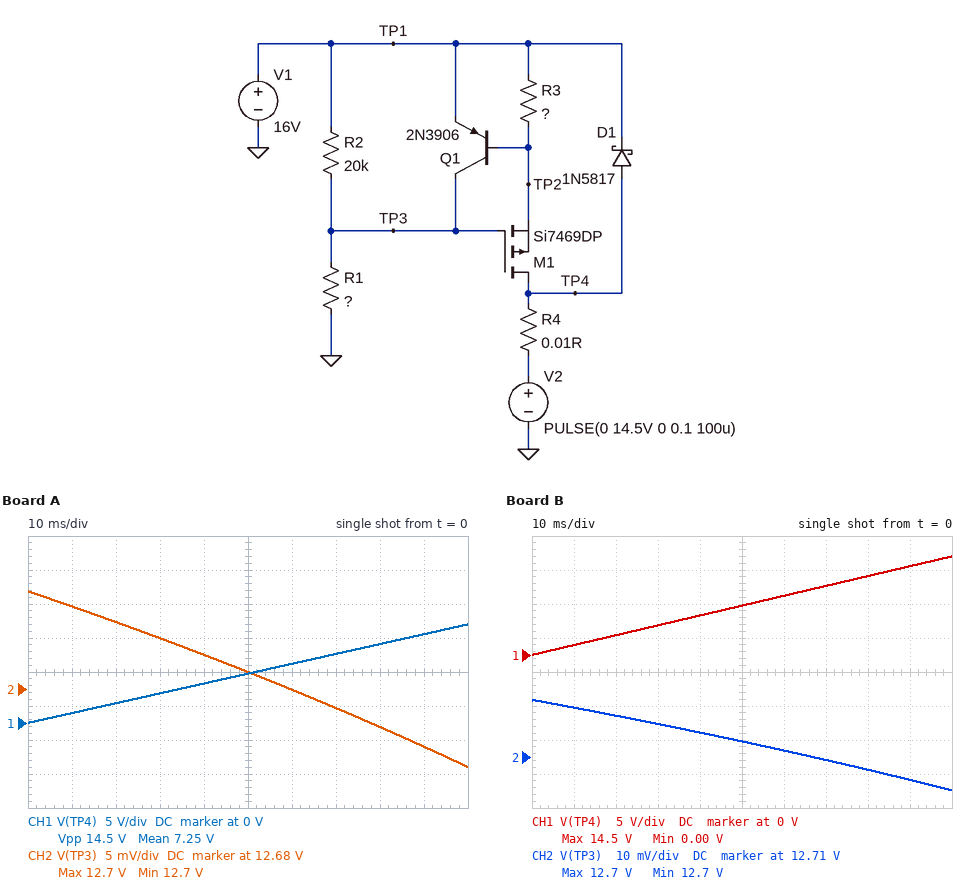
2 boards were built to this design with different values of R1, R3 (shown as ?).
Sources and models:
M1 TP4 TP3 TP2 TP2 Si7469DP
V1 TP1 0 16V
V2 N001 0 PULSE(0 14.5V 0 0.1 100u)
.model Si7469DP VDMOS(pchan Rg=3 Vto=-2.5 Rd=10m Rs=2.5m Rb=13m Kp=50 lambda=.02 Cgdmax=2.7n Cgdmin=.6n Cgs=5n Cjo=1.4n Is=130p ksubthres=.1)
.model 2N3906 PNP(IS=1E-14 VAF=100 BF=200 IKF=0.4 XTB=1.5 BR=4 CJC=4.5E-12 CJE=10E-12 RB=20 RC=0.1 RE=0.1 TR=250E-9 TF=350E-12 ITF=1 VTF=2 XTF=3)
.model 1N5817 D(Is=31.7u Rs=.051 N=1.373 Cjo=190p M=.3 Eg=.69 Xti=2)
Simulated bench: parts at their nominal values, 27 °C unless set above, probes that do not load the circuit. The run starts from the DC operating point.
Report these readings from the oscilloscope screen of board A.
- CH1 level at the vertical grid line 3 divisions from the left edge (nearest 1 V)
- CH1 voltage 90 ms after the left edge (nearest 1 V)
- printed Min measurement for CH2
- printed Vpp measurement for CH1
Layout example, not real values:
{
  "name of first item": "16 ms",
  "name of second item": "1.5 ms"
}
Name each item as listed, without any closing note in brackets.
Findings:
{
  "CH1 level at the vertical grid line 3 divisions from the left edge": "4 V",
  "CH1 voltage 90 ms after the left edge": "13 V",
  "printed Min measurement for CH2": "12.7 V",
  "printed Vpp measurement for CH1": "14.5 V"
}
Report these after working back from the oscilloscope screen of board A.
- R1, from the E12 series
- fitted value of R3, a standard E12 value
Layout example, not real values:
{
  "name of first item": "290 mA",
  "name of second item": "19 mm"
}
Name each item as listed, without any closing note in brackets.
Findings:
{
  "R1, from the E12 series": "6.8 kΩ",
  "fitted value of R3, a standard E12 value": "0.82 Ω"
}
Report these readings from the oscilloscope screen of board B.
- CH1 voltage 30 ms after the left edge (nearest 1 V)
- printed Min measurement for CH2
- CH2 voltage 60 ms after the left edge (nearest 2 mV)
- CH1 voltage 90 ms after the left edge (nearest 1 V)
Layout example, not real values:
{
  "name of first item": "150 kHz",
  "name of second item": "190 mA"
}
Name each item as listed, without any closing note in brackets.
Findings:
{
  "CH1 voltage 30 ms after the left edge": "4 V",
  "printed Min measurement for CH2": "12.7 V",
  "CH2 voltage 60 ms after the left edge": "12.712 V",
  "CH1 voltage 90 ms after the left edge": "13 V"
}
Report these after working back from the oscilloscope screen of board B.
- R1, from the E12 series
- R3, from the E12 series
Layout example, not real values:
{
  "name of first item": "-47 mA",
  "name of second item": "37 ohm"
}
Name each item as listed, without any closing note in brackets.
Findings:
{
  "R1, from the E12 series": "27 kΩ",
  "R3, from the E12 series": "0.68 Ω"
}
